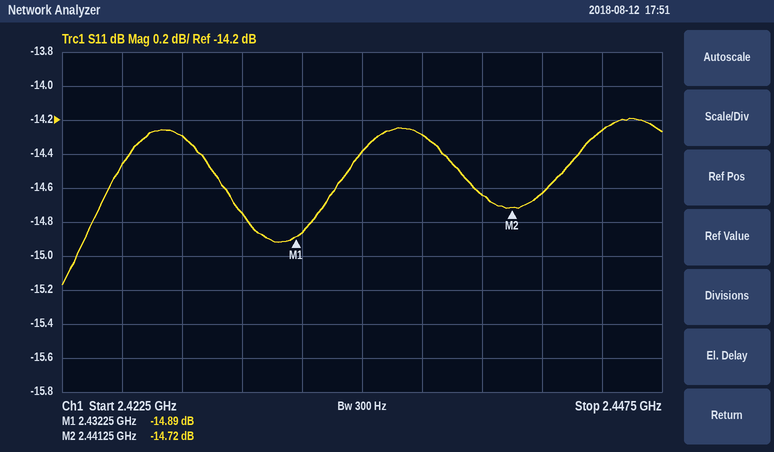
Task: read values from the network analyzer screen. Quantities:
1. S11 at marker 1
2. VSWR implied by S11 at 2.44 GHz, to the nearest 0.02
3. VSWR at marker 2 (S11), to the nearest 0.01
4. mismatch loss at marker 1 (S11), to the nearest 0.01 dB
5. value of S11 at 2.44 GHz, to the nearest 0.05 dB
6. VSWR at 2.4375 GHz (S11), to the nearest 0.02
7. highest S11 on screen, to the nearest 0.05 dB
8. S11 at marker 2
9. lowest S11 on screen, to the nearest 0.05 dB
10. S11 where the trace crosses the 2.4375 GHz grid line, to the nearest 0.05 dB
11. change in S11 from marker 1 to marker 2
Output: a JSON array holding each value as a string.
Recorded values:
["-14.89 dB", "1.46", "1.45", "0.14 dB", "-14.65 dB", "1.48", "-14.20 dB", "-14.72 dB", "-15.15 dB", "-14.30 dB", "0.17 dB"]
